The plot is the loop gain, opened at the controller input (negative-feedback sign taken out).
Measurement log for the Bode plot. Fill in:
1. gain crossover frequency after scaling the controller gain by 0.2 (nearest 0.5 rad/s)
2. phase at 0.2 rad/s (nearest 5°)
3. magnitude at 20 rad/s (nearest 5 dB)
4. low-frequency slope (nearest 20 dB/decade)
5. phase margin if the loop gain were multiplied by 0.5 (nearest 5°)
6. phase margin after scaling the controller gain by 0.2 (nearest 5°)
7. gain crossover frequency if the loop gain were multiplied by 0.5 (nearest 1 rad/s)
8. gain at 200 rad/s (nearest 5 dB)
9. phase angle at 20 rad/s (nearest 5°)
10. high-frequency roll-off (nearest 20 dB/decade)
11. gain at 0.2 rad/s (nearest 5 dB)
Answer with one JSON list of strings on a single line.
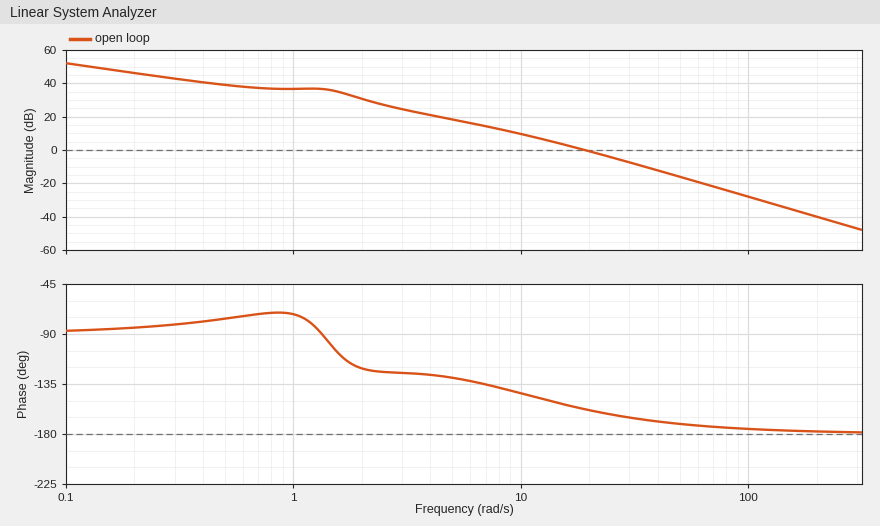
["7.0 rad/s", "-85°", "0 dB", "-20 dB/decade", "30°", "45°", "13 rad/s", "-40 dB", "-160°", "-40 dB/decade", "45 dB"]
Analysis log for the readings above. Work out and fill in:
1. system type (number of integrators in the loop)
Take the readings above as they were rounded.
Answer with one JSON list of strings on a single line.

["1"]
